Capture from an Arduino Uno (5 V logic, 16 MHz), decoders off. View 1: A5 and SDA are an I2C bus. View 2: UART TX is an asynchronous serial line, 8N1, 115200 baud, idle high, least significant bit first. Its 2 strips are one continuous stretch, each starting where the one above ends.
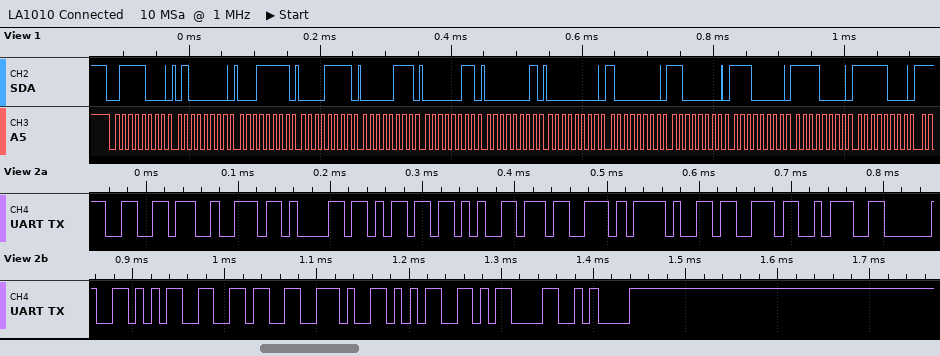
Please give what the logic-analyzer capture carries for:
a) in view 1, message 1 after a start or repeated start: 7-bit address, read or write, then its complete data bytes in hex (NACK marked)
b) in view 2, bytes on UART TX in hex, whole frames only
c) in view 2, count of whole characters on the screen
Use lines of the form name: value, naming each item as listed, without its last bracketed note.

in view 1, message 1 after a start or repeated start: 7-bit address, read or write, then its complete data bytes in hex: 0x3C write: 40 1F 0F 07 03 01 00 80 C0 E0 F0 F8
in view 2, bytes on UART TX in hex, whole frames only: 66 72 61 6D 65 73 2F 73 3A 20 35 36 2E 35 0D 0A
in view 2, count of whole characters on the screen: 16
